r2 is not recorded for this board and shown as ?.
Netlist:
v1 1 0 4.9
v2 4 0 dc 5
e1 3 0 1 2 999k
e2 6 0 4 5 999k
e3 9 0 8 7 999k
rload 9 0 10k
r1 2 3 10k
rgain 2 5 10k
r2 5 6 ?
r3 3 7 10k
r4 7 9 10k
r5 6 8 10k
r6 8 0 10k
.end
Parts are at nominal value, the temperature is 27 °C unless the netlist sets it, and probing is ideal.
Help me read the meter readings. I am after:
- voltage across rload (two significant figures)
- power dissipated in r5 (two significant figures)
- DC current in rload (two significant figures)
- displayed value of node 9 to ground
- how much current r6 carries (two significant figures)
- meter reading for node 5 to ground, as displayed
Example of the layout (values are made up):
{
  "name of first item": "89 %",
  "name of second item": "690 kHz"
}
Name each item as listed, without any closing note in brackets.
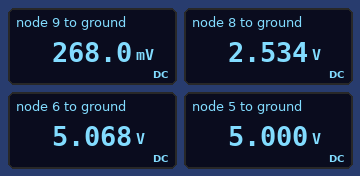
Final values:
{
  "voltage across rload": "270 mV",
  "power dissipated in r5": "640 µW",
  "DC current in rload": "27 µA",
  "displayed value of node 9 to ground": "268.0 mV",
  "how much current r6 carries": "250 µA",
  "meter reading for node 5 to ground, as displayed": "5.000 V"
}
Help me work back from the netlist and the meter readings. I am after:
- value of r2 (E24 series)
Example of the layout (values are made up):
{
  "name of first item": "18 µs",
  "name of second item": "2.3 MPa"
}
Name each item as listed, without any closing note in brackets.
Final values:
{
  "value of r2": "6.8 kΩ"
}
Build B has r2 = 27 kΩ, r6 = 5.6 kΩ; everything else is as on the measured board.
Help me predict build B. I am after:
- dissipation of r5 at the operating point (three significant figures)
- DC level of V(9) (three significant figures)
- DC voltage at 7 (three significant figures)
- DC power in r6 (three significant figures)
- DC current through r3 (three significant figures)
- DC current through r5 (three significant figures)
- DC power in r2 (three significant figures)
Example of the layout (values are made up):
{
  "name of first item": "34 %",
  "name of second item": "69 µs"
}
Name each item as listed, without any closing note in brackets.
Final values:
{
  "dissipation of r5 at the operating point": "1.14 mW",
  "DC level of V(9)": "-1.02 V",
  "DC voltage at 7": "1.89 V",
  "DC power in r6": "639 µW",
  "DC current through r3": "291 µA",
  "DC current through r5": "338 µA",
  "DC power in r2": "2.70 µW"
}
